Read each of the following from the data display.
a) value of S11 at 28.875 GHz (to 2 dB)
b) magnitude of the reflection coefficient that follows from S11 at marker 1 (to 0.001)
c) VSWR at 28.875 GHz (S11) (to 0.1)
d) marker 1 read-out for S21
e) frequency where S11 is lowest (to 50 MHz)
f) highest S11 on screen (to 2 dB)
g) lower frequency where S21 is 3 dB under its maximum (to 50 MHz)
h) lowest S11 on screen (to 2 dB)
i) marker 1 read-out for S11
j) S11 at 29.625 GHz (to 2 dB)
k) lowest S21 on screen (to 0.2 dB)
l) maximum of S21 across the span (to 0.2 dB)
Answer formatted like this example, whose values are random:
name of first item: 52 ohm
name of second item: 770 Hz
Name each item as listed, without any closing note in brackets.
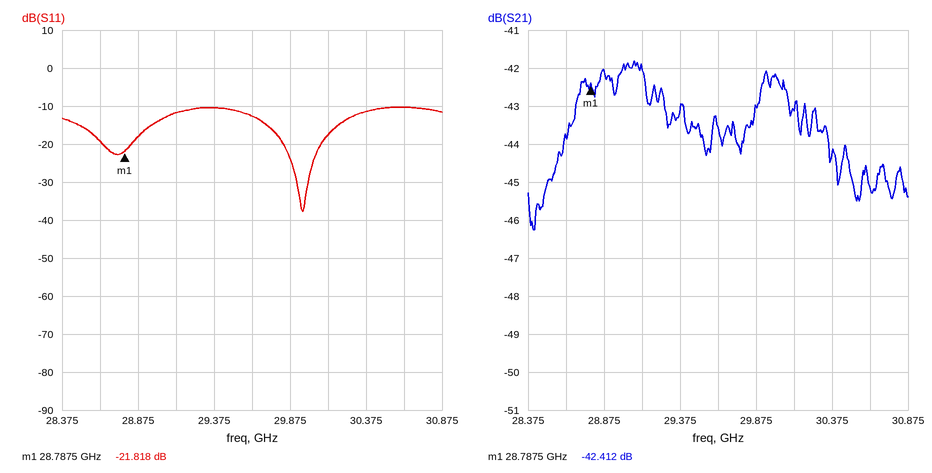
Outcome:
value of S11 at 28.875 GHz: -18 dB
magnitude of the reflection coefficient that follows from S11 at marker 1: 0.081
VSWR at 28.875 GHz (S11): 1.3
marker 1 read-out for S21: -42.412 dB
frequency where S11 is lowest: 29.95 GHz
highest S11 on screen: -10 dB
lower frequency where S21 is 3 dB under its maximum: 28.55 GHz
lowest S11 on screen: -38 dB
marker 1 read-out for S11: -21.818 dB
S11 at 29.625 GHz: -12 dB
lowest S21 on screen: -46.2 dB
maximum of S21 across the span: -41.8 dB
